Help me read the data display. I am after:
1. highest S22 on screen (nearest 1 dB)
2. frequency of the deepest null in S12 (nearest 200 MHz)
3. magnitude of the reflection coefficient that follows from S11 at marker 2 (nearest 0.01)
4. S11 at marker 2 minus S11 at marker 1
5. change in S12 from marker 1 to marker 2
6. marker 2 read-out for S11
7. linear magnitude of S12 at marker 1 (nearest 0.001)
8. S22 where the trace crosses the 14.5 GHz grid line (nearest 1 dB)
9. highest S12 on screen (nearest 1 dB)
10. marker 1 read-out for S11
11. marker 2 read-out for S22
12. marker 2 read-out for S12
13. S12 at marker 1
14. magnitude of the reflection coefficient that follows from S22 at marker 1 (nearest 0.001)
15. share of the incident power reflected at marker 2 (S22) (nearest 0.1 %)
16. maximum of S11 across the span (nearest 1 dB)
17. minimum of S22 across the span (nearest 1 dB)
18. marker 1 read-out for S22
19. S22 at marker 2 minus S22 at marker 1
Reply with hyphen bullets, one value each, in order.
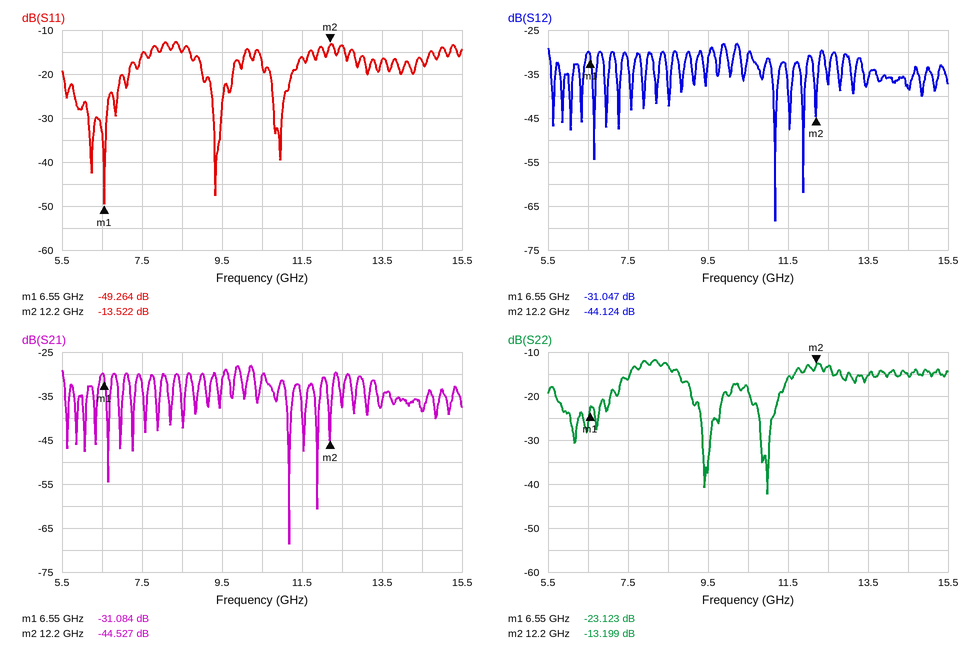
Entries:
- -12 dB
- 11.2 GHz
- 0.21
- 35.742 dB
- -13.077 dB
- -13.522 dB
- 0.028
- -15 dB
- -28 dB
- -49.264 dB
- -13.199 dB
- -44.124 dB
- -31.047 dB
- 0.070
- 4.8 %
- -13 dB
- -42 dB
- -23.123 dB
- 9.924 dB
